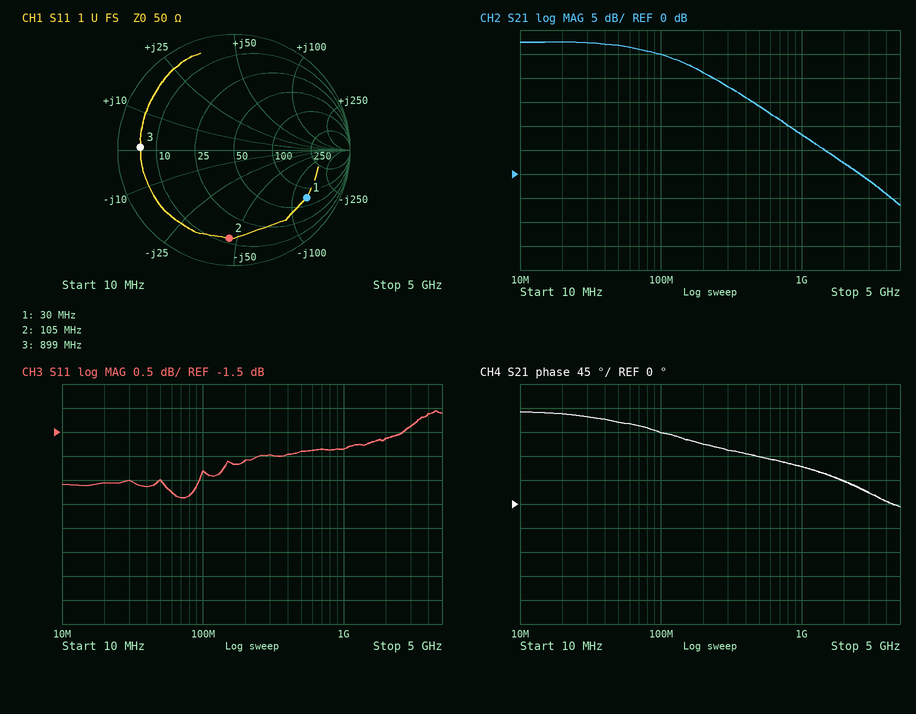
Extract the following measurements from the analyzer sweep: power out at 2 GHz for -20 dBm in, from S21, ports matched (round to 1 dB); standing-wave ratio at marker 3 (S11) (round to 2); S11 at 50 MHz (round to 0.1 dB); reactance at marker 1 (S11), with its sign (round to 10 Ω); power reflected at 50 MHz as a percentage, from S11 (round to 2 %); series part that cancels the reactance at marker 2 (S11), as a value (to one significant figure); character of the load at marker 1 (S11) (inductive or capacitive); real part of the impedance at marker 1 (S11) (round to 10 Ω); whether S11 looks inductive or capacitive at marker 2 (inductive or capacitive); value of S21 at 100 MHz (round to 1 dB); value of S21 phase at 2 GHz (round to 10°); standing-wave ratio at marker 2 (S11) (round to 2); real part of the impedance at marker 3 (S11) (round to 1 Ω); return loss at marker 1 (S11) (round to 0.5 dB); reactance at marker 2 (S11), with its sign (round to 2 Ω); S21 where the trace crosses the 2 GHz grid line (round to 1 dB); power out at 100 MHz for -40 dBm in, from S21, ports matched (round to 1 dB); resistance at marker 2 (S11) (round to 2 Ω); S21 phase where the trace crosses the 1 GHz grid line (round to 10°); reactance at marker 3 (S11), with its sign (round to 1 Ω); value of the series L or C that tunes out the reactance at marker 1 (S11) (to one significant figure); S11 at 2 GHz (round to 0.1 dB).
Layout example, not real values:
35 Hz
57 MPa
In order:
-18 dBm
10
-2.5 dB
-130 Ω
56 %
70 nH
capacitive
70 Ω
capacitive
25 dB
40°
8
5 Ω
2.5 dB
-46 Ω
2 dB
-15 dBm
12 Ω
70°
+1 Ω
700 nH
-1.6 dB
